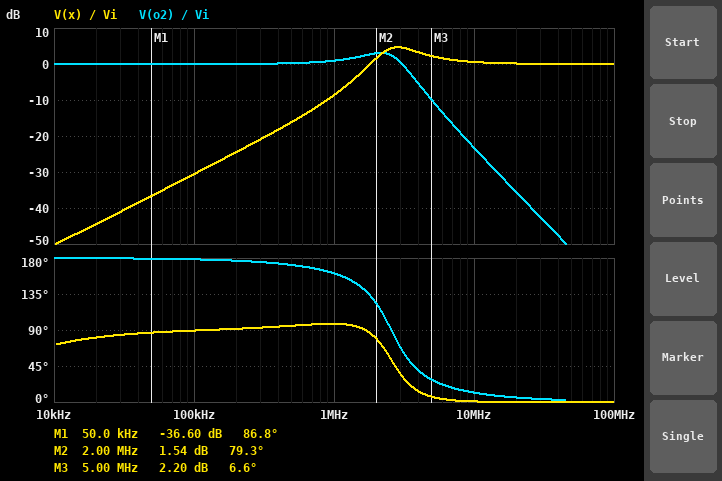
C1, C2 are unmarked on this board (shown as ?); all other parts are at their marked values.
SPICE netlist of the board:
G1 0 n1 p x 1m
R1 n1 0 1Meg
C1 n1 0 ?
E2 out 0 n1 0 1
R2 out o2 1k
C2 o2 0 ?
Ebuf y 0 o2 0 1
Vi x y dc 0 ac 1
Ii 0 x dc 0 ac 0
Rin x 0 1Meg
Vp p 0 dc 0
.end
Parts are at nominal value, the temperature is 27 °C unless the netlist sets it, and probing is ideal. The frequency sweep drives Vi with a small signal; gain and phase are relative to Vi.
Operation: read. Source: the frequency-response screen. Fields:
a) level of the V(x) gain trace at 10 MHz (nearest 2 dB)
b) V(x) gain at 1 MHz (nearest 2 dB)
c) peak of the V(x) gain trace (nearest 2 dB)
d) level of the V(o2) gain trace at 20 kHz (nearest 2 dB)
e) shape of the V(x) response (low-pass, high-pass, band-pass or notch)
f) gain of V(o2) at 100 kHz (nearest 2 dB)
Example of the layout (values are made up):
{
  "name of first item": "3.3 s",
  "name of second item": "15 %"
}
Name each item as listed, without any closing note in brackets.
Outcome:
{
  "level of the V(x) gain trace at 10 MHz": "0 dB",
  "V(x) gain at 1 MHz": "-8 dB",
  "peak of the V(x) gain trace": "4 dB",
  "level of the V(o2) gain trace at 20 kHz": "0 dB",
  "shape of the V(x) response": "high-pass",
  "gain of V(o2) at 100 kHz": "0 dB"
}
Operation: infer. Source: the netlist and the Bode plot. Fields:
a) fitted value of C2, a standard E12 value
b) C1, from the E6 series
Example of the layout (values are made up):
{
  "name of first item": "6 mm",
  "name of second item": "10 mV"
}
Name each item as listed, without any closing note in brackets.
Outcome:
{
  "fitted value of C2, a standard E12 value": "82 pF",
  "C1, from the E6 series": "47 pF"
}
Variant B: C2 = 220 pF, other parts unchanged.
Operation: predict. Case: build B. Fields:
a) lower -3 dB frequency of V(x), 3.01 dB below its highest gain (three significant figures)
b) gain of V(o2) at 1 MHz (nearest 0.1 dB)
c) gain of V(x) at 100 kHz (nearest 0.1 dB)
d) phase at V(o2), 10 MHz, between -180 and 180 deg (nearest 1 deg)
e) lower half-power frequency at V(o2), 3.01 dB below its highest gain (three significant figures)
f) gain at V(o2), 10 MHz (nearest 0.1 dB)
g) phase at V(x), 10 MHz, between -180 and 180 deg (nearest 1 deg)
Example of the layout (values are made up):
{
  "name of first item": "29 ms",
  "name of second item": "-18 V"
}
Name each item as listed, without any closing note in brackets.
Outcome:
{
  "lower -3 dB frequency of V(x), 3.01 dB below its highest gain": "1.33 MHz",
  "gain of V(o2) at 1 MHz": "3.6 dB",
  "gain of V(x) at 100 kHz": "-30.5 dB",
  "phase at V(o2), 10 MHz, between -180 and 180 deg": "4 deg",
  "lower half-power frequency at V(o2), 3.01 dB below its highest gain": "1.04 MHz",
  "gain at V(o2), 10 MHz": "-32.0 dB",
  "phase at V(x), 10 MHz, between -180 and 180 deg": "0 deg"
}
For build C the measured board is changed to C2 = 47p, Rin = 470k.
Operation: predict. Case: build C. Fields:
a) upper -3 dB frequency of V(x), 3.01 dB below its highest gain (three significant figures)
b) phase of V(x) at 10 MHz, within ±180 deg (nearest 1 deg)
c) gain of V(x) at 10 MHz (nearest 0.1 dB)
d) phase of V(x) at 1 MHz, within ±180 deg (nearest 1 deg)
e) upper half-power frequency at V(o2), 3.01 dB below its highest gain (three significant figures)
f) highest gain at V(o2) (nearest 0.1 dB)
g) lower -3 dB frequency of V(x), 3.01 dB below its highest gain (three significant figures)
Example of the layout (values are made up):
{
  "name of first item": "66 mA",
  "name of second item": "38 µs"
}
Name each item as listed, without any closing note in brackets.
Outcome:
{
  "upper -3 dB frequency of V(x), 3.01 dB below its highest gain": "17.5 MHz",
  "phase of V(x) at 10 MHz, within ±180 deg": "2 deg",
  "gain of V(x) at 10 MHz": "0.9 dB",
  "phase of V(x) at 1 MHz, within ±180 deg": "88 deg",
  "upper half-power frequency at V(o2), 3.01 dB below its highest gain": "3.96 MHz",
  "highest gain at V(o2)": "1.2 dB",
  "lower -3 dB frequency of V(x), 3.01 dB below its highest gain": "2.46 MHz"
}
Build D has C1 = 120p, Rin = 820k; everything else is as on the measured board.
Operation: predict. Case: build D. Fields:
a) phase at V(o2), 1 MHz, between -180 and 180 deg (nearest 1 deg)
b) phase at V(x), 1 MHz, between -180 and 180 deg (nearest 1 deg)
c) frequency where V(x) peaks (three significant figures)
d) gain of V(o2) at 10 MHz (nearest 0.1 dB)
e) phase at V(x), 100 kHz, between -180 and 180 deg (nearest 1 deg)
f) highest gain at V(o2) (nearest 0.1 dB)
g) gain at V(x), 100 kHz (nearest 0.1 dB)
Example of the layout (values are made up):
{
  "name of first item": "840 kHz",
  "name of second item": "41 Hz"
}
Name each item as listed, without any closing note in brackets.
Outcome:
{
  "phase at V(o2), 1 MHz, between -180 and 180 deg": "129 deg",
  "phase at V(x), 1 MHz, between -180 and 180 deg": "66 deg",
  "frequency where V(x) peaks": "1.96 MHz",
  "gain of V(o2) at 10 MHz": "-31.7 dB",
  "phase at V(x), 100 kHz, between -180 and 180 deg": "88 deg",
  "highest gain at V(o2)": "0.3 dB",
  "gain at V(x), 100 kHz": "-22.4 dB"
}
